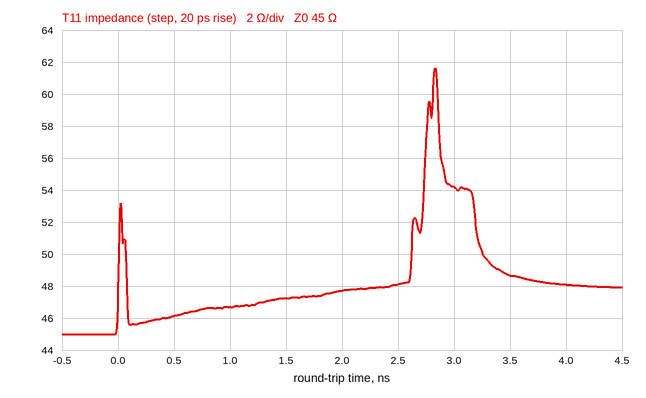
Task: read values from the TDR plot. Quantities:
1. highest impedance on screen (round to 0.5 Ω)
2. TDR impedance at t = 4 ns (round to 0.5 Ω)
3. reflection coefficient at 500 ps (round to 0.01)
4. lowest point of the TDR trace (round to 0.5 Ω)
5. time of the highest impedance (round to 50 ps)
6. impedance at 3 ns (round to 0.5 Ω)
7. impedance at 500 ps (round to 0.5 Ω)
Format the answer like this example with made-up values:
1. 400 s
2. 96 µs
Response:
1. 61.5 Ω
2. 48.0 Ω
3. +0.01
4. 45.0 Ω
5. 2.85 ns
6. 54.0 Ω
7. 46.0 Ω
